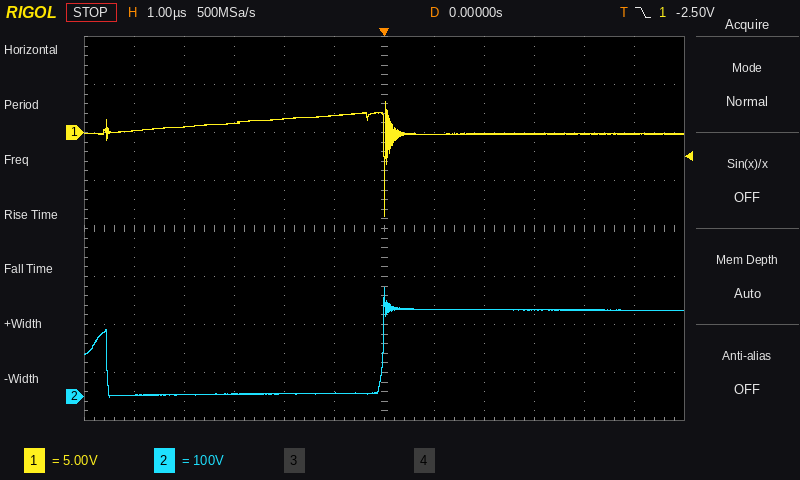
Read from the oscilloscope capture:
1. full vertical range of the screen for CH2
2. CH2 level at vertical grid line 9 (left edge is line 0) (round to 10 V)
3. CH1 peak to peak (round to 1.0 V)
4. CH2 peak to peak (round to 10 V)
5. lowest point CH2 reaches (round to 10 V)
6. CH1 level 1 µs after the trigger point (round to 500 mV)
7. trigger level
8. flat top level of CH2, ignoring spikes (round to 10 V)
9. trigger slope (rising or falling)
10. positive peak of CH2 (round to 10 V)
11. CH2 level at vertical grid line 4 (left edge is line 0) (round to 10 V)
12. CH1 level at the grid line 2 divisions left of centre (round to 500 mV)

800 V
180 V
12.0 V
230 V
0 V
0.0 V
-2.50 V
180 V
falling
230 V
10 V
1.5 V
